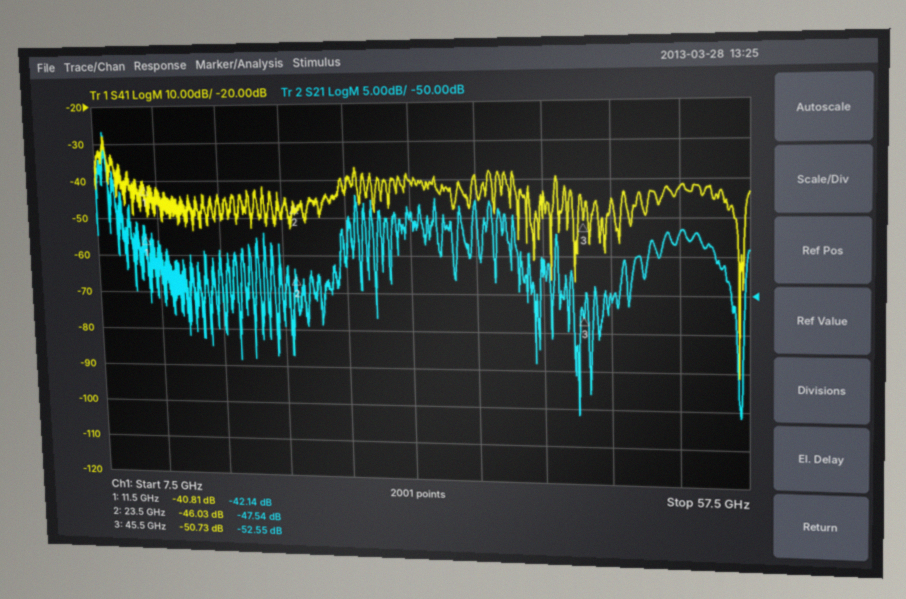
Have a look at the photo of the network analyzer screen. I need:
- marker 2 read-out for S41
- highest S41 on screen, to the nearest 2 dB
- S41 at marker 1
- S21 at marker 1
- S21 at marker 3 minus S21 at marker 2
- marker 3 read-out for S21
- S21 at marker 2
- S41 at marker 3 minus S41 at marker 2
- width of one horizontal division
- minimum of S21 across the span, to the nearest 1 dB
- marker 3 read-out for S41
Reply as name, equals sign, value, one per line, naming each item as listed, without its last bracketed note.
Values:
marker 2 read-out for S41 = -46.03 dB
highest S41 on screen, to the nearest 2 dB = -28 dB
S41 at marker 1 = -40.81 dB
S21 at marker 1 = -42.14 dB
S21 at marker 3 minus S21 at marker 2 = -5.01 dB
marker 3 read-out for S21 = -52.55 dB
S21 at marker 2 = -47.54 dB
S41 at marker 3 minus S41 at marker 2 = -4.70 dB
width of one horizontal division = 5 GHz
minimum of S21 across the span, to the nearest 1 dB = -66 dB
marker 3 read-out for S41 = -50.73 dB
